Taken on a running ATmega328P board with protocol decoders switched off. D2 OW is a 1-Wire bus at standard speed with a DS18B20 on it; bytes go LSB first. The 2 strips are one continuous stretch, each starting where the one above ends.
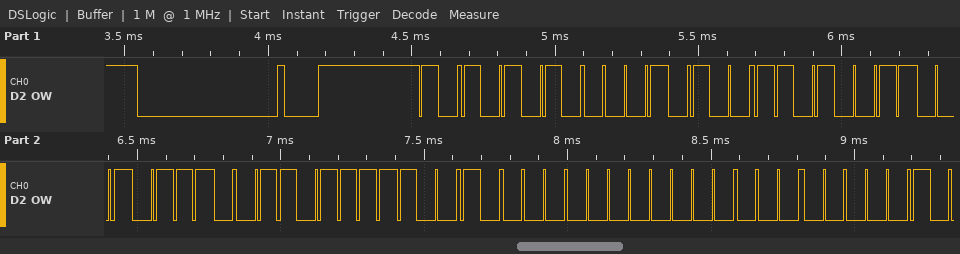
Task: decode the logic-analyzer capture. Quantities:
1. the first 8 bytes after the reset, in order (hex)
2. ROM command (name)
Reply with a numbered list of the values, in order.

1. 55 28 CB 74 F6 09 00 00
2. Match ROM
